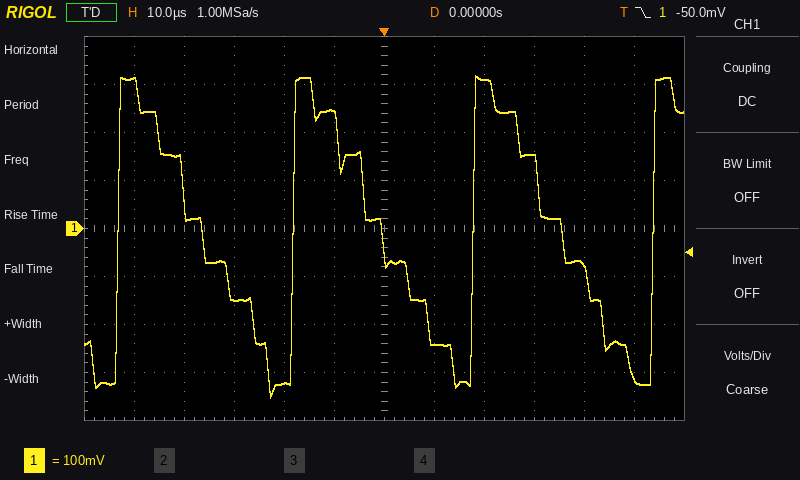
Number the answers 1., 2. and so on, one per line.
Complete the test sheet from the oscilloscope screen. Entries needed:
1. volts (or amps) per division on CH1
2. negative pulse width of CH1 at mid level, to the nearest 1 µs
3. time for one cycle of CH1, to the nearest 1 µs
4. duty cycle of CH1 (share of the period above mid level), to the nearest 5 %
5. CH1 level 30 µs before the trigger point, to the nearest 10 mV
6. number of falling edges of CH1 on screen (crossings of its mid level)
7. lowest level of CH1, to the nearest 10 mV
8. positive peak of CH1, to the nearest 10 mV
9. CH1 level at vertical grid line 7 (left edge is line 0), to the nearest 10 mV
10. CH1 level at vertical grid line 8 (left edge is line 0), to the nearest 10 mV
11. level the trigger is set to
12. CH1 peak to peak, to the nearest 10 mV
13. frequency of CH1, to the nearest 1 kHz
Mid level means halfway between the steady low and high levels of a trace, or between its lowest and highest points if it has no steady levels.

1. 100 mV
2. 18 µs
3. 36 µs
4. 50 %
5. -150 mV
6. 3
7. -350 mV
8. 320 mV
9. -240 mV
10. 310 mV
11. -50.0 mV
12. 670 mV
13. 28 kHz
